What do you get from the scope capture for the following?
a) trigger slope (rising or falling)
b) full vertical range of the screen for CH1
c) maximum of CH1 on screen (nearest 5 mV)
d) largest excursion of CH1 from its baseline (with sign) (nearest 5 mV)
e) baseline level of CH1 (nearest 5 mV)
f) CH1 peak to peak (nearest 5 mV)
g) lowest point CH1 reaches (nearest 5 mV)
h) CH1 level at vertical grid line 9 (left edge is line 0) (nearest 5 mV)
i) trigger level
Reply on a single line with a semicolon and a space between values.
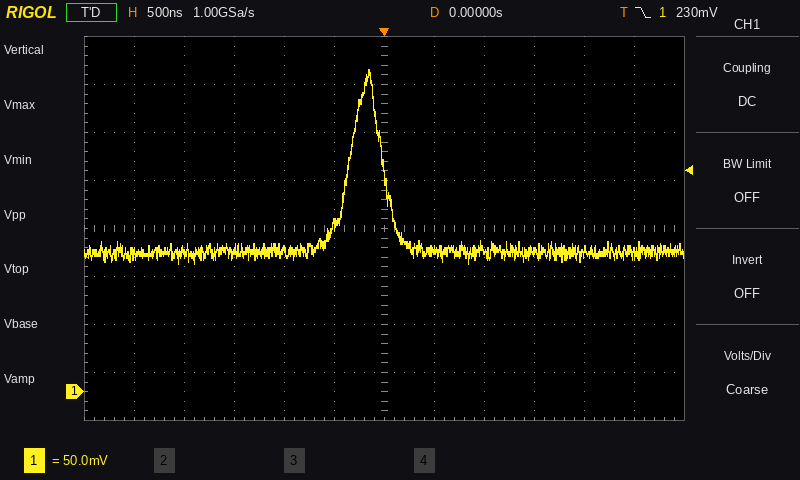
falling; 400 mV; 335 mV; +190 mV; 145 mV; 200 mV; 135 mV; 145 mV; 230 mV
